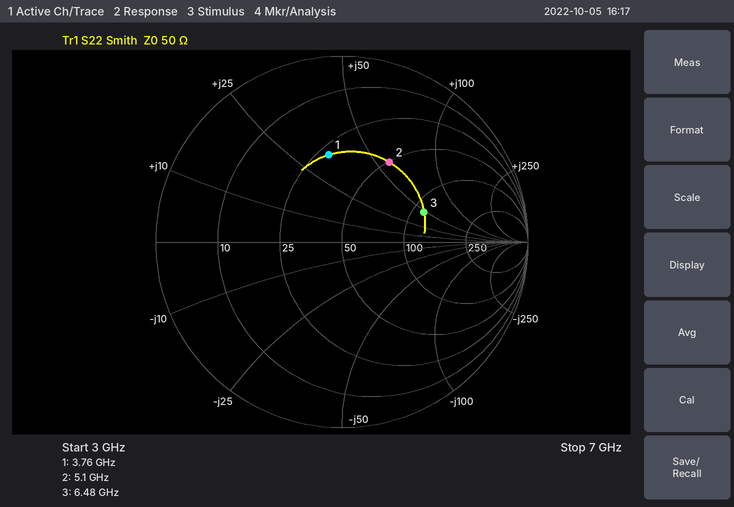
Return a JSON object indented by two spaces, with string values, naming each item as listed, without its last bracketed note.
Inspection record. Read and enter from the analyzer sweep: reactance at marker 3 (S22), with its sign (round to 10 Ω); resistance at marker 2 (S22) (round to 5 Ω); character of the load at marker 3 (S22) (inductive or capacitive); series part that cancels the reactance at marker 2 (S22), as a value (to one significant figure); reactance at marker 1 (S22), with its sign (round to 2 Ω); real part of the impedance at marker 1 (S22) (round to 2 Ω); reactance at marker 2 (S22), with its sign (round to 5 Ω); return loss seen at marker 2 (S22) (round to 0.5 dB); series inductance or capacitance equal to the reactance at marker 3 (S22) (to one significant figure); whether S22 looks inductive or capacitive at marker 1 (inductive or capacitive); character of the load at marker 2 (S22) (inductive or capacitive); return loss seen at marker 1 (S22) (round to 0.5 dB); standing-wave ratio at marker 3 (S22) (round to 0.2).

{
  "reactance at marker 3 (S22), with its sign": "+50 Ω",
  "resistance at marker 2 (S22)": "50 Ω",
  "character of the load at marker 3 (S22)": "inductive",
  "series part that cancels the reactance at marker 2 (S22), as a value": "500 fF",
  "reactance at marker 1 (S22), with its sign": "+34 Ω",
  "real part of the impedance at marker 1 (S22)": "28 Ω",
  "reactance at marker 2 (S22), with its sign": "+60 Ω",
  "return loss seen at marker 2 (S22)": "6.0 dB",
  "series inductance or capacitance equal to the reactance at marker 3 (S22)": "1 nH",
  "whether S22 looks inductive or capacitive at marker 1": "inductive",
  "character of the load at marker 2 (S22)": "inductive",
  "return loss seen at marker 1 (S22)": "6.5 dB",
  "standing-wave ratio at marker 3 (S22)": "2.8"
}
